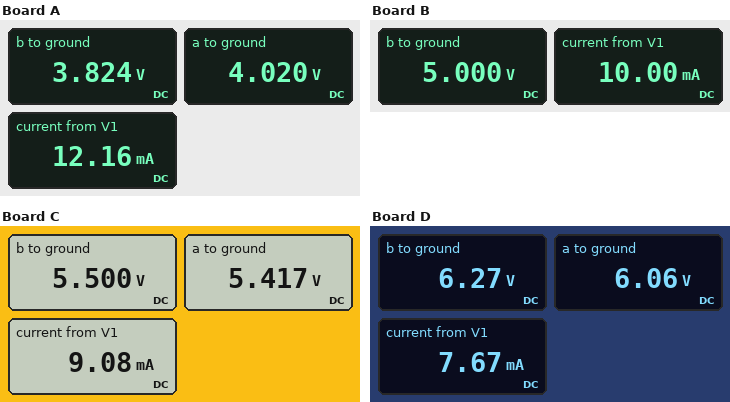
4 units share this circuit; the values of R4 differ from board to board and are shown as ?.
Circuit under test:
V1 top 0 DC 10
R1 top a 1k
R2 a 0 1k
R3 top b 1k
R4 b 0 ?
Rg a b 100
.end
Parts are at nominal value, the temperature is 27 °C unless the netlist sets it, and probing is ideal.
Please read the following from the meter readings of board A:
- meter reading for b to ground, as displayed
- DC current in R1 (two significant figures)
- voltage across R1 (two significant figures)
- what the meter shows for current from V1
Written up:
3.824 V
6.0 mA
6.0 V
12.16 mA
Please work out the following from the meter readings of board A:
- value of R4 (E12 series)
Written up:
470 Ω
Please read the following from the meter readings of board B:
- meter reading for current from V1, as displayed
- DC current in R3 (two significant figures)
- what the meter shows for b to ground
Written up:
10.00 mA
5.0 mA
5.000 V
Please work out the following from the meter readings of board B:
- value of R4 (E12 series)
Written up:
1 kΩ
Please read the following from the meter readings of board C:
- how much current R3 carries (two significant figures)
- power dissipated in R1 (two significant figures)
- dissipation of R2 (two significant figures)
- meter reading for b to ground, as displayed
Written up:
4.5 mA
21 mW
29 mW
5.500 V
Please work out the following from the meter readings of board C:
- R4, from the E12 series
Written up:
1.5 kΩ
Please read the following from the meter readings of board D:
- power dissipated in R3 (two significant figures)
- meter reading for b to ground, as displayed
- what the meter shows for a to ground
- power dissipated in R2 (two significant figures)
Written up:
14 mW
6.27 V
6.06 V
37 mW
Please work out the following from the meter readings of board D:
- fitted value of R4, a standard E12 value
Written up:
3.9 kΩ
